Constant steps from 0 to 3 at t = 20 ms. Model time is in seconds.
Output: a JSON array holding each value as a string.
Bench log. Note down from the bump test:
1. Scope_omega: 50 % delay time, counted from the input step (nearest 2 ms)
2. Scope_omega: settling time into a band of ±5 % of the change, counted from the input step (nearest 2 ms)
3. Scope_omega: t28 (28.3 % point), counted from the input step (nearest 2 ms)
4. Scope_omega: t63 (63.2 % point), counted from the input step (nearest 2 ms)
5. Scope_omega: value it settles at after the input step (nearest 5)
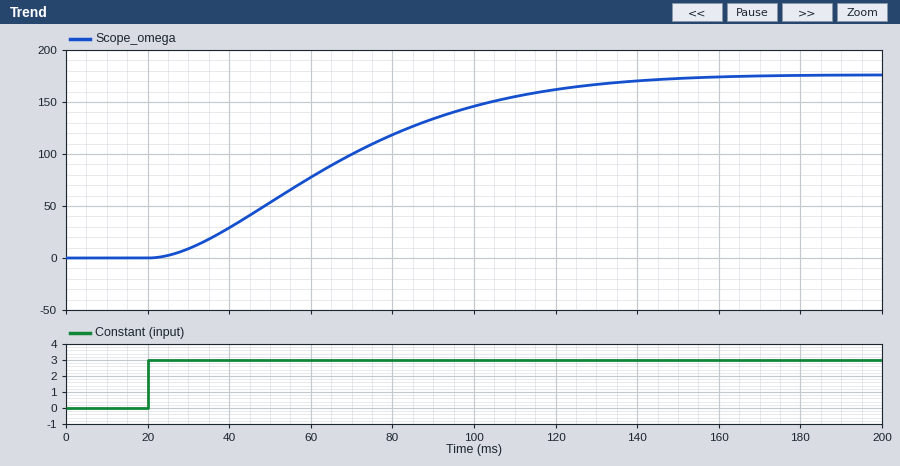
["44 ms", "110 ms", "28 ms", "56 ms", "175"]
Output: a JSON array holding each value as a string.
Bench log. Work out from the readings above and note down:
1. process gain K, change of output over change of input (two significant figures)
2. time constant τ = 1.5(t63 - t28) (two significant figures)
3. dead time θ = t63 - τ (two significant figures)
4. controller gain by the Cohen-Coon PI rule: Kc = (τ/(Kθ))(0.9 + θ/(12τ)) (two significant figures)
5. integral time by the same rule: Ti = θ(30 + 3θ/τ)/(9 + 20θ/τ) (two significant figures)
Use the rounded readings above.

["58", "42 ms", "14 ms", "0.048", "28 ms"]
